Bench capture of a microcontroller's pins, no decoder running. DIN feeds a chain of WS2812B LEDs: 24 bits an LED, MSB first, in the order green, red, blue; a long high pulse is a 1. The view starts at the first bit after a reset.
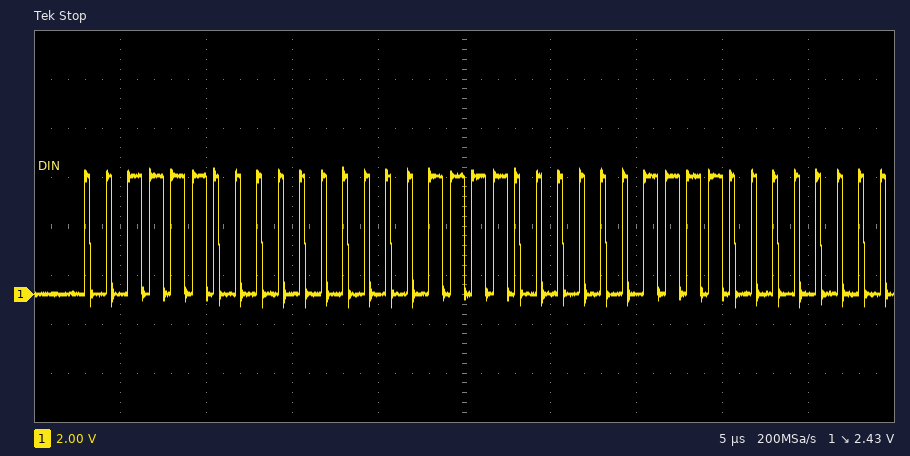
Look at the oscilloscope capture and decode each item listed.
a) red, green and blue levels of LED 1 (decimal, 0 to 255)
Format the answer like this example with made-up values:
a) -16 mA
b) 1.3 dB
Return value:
a) 0, 60, 240
